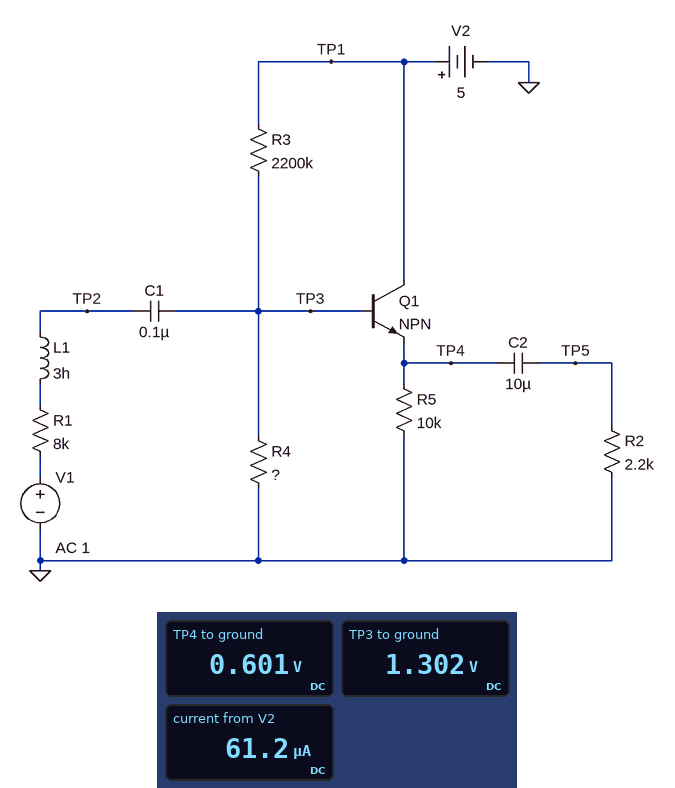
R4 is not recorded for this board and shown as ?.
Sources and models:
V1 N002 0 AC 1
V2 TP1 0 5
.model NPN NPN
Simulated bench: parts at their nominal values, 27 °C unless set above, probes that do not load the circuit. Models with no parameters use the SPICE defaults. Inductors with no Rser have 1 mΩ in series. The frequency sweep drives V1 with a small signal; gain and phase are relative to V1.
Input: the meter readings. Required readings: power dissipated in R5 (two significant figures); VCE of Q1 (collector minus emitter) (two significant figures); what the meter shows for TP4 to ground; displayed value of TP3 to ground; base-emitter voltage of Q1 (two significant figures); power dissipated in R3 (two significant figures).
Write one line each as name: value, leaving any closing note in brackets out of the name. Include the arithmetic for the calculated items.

power dissipated in R5: (601 mV)^2 / 10 kΩ = 36 µW
VCE of Q1 (collector minus emitter): 5 V - 601 mV = 4.4 V
what the meter shows for TP4 to ground: 0.601 V
displayed value of TP3 to ground: 1.302 V
base-emitter voltage of Q1: 1.302 V - 601 mV = 700 mV
power dissipated in R3: (5 V - 1.302 V)^2 / 2.2 MΩ = 6.2 µW
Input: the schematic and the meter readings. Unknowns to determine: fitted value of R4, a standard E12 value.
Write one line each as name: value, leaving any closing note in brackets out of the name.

fitted value of R4, a standard E12 value: 1.2 MΩ
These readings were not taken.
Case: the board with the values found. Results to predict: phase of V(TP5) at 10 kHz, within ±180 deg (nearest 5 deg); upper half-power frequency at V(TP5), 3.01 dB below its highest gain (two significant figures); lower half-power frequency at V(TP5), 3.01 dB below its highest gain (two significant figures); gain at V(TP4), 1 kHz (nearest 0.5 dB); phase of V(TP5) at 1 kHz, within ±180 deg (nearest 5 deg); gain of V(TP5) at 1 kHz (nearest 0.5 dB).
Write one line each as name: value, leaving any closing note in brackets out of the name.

phase of V(TP5) at 10 kHz, within ±180 deg: -45 deg
upper half-power frequency at V(TP5), 3.01 dB below its highest gain: 9.7 kHz
lower half-power frequency at V(TP5), 3.01 dB below its highest gain: 13 Hz
gain at V(TP4), 1 kHz: -2.5 dB
phase of V(TP5) at 1 kHz, within ±180 deg: -5 deg
gain of V(TP5) at 1 kHz: -2.5 dB
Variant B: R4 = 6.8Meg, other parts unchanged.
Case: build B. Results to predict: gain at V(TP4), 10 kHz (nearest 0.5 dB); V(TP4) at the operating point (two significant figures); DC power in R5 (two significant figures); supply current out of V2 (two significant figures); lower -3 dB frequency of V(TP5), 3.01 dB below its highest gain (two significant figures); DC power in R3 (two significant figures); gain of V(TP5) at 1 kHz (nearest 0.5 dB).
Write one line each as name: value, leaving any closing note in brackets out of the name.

gain at V(TP4), 10 kHz: -4.5 dB
V(TP4) at the operating point: 1.2 V
DC power in R5: 130 µW
supply current out of V2: 120 µA
lower -3 dB frequency of V(TP5), 3.01 dB below its highest gain: 14 Hz
DC power in R3: 4.4 µW
gain of V(TP5) at 1 kHz: -1.5 dB
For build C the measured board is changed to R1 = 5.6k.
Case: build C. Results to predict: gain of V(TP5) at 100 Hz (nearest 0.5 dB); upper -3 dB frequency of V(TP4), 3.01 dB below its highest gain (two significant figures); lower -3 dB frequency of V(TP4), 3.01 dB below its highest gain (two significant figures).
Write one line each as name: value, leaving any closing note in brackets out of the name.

gain of V(TP5) at 100 Hz: -2.0 dB
upper -3 dB frequency of V(TP4), 3.01 dB below its highest gain: 9.6 kHz
lower -3 dB frequency of V(TP4), 3.01 dB below its highest gain: 8.8 Hz
